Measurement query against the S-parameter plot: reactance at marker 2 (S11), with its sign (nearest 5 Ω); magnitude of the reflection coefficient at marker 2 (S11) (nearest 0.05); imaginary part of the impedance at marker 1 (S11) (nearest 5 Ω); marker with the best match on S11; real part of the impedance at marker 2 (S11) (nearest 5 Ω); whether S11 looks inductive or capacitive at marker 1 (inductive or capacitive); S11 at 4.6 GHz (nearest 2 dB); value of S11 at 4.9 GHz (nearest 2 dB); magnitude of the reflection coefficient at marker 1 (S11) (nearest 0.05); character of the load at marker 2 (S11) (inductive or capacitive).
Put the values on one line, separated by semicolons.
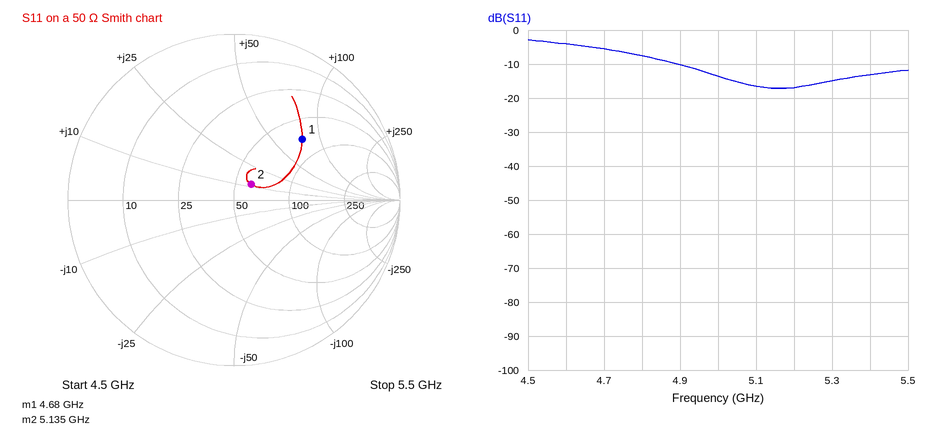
+10 Ω; 0.15; +75 Ω; marker 2; 60 Ω; inductive; -4 dB; -10 dB; 0.55; inductive
